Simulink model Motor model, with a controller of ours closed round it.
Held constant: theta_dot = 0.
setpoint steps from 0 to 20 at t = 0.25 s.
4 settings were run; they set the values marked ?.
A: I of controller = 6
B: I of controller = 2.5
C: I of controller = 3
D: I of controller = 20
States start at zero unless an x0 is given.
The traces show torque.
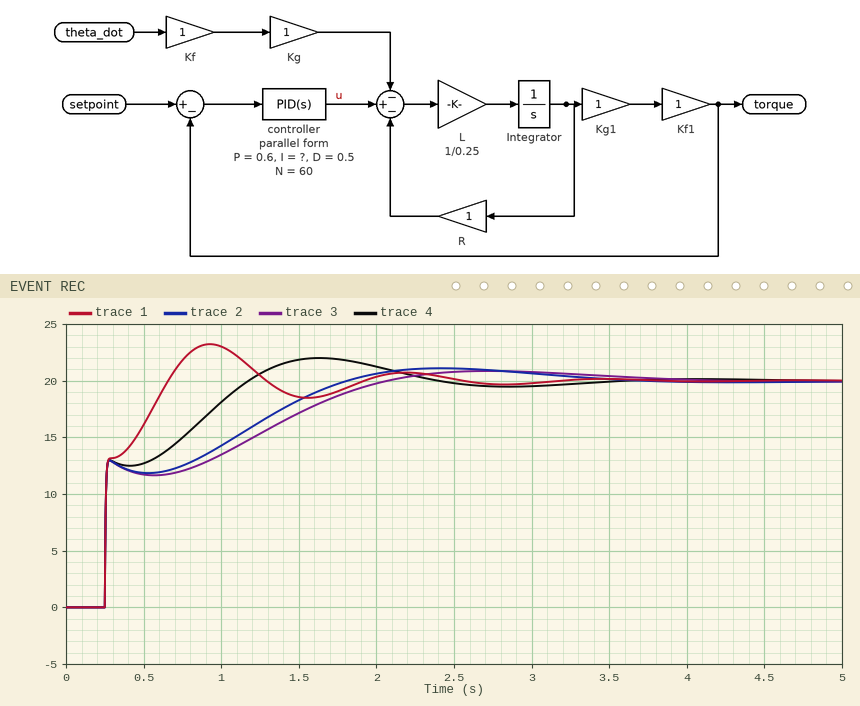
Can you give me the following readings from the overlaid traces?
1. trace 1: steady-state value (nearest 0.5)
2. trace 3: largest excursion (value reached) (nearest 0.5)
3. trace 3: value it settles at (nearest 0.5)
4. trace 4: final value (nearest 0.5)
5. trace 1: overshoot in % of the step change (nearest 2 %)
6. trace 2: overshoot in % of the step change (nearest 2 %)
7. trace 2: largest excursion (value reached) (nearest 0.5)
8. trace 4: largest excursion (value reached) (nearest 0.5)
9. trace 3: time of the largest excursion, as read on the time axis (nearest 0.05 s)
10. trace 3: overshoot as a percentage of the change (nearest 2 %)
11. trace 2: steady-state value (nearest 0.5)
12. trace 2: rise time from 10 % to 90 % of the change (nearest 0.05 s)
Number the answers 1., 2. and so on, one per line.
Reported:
1. 20.0
2. 21.0
3. 20.0
4. 20.0
5. 16 %
6. 6 %
7. 21.0
8. 22.0
9. 2.70 s
10. 4 %
11. 20.0
12. 1.20 s
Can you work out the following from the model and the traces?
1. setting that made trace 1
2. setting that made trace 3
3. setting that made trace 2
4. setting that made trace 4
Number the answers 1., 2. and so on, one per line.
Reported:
1. D
2. B
3. C
4. A
